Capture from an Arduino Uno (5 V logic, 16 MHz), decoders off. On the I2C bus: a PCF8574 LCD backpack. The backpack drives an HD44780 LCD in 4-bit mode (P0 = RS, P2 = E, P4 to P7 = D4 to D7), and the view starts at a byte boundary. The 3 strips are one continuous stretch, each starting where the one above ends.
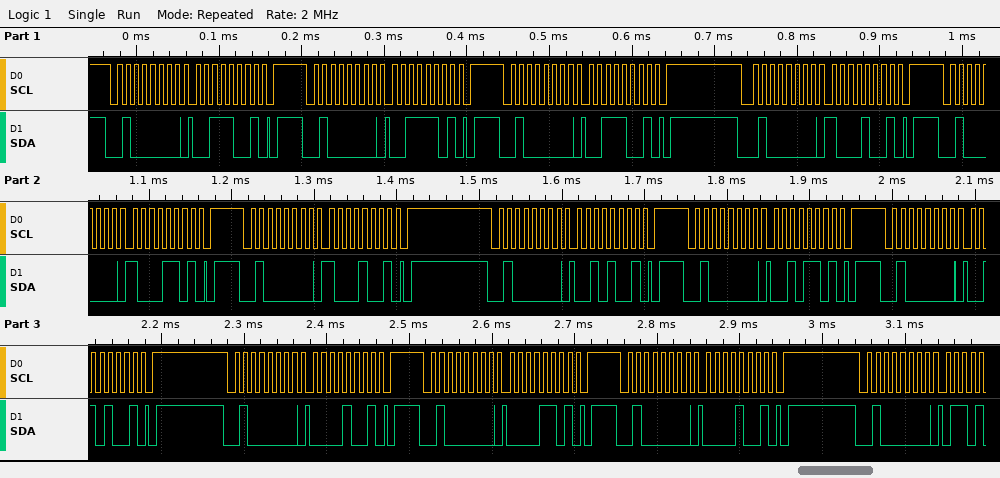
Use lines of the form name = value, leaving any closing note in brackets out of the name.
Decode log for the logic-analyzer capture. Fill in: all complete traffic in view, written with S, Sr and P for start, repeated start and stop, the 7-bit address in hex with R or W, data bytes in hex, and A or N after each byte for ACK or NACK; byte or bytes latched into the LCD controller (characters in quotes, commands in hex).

all complete traffic in view, written with S, Sr and P for start, repeated start and stop, the 7-bit address in hex with R or W, data bytes in hex, and A or N after each byte for ACK or NACK = S 20W A 39 A P S 20W A 3D A P S 20W A 39 A P S 20W A 89 A P S 20W A 8D A P S 20W A 89 A P S 20W A 29 A P S 20W A 2D A P S 20W A 29 A P S 20W A 09 A P S 20W A 0D A P S 20W A 09 A P S 20W A
byte or bytes latched into the LCD controller = '8' ' '
